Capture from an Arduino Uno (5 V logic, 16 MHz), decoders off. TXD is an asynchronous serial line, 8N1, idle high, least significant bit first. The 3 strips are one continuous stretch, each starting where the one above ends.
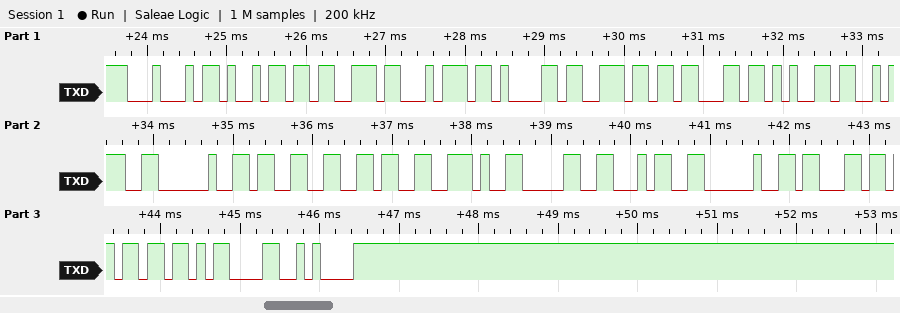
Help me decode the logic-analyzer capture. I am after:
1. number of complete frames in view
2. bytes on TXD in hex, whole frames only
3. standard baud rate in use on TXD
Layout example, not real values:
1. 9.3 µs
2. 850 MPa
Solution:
1. 20
2. 44 69 73 74 61 6E 63 65 3A 20 33 36 2E 30 34 20 63 6D 0D 0A
3. 9600 baud
